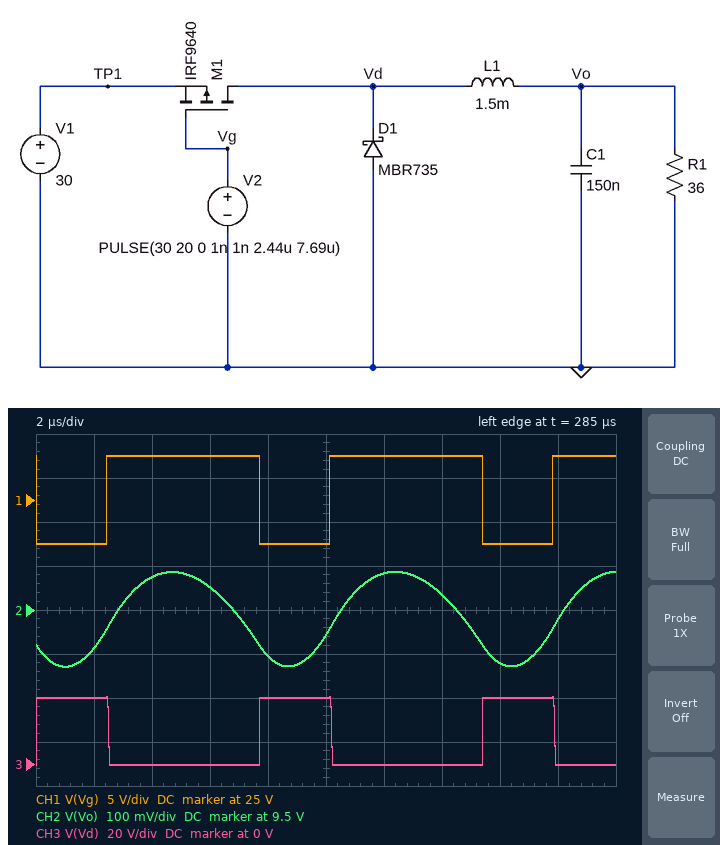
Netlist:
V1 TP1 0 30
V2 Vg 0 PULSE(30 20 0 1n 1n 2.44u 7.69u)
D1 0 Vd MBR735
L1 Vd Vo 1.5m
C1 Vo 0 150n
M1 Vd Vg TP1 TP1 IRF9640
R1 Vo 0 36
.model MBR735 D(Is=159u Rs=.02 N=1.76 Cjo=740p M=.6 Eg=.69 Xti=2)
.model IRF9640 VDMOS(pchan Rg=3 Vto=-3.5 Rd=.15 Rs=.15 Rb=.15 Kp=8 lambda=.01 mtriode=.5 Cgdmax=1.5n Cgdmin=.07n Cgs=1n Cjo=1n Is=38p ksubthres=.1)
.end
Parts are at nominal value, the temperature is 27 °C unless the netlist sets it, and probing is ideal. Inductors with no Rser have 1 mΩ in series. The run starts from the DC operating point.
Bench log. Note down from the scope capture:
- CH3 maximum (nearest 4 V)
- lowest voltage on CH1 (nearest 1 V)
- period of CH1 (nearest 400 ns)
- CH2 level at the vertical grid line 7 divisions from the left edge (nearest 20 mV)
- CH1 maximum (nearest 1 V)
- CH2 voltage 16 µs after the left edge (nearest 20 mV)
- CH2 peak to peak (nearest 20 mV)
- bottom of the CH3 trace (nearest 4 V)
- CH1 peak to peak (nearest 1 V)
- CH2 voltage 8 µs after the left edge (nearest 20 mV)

32 V
20 V
7.6 µs
9.54 V
30 V
9.38 V
220 mV
0 V
10 V
9.40 V
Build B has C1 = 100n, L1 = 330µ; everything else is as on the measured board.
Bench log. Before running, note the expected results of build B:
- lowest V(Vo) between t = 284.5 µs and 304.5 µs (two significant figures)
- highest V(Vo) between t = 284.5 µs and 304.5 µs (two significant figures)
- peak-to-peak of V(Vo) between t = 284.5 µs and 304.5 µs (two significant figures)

8.6 V
10 V
1.5 V
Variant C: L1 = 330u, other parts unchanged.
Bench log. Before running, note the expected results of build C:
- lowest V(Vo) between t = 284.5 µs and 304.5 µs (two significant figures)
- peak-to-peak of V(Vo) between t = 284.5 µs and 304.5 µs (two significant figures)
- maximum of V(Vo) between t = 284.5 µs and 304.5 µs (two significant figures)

8.9 V
1.0 V
9.9 V
